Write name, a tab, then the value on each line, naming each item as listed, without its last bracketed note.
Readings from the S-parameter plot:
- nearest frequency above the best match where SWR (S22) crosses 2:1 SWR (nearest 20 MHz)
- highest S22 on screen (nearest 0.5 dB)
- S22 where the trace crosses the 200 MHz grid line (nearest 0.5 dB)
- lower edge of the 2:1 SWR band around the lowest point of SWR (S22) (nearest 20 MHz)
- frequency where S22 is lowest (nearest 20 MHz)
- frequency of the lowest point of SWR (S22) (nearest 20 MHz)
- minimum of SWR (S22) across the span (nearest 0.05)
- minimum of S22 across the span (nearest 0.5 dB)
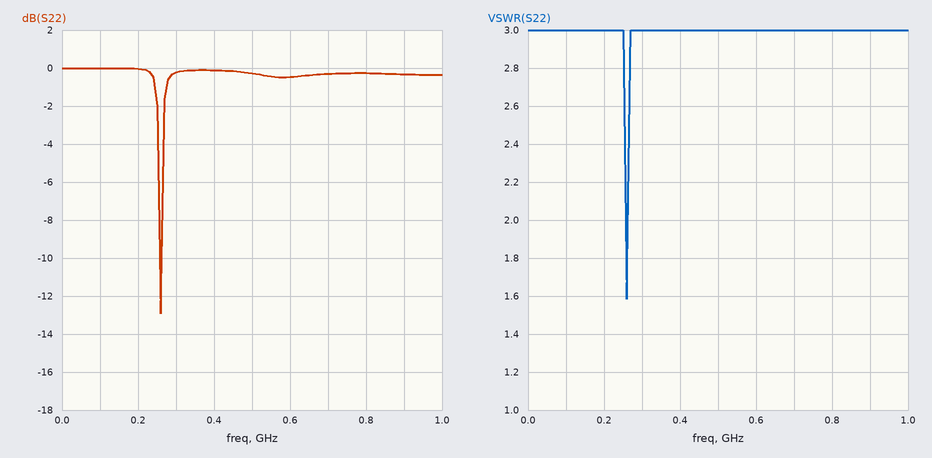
nearest frequency above the best match where SWR (S22) crosses 2:1 SWR	260 MHz
highest S22 on screen	0.0 dB
S22 where the trace crosses the 200 MHz grid line	0.0 dB
lower edge of the 2:1 SWR band around the lowest point of SWR (S22)	260 MHz
frequency where S22 is lowest	260 MHz
frequency of the lowest point of SWR (S22)	260 MHz
minimum of SWR (S22) across the span	1.60
minimum of S22 across the span	-13.0 dB
